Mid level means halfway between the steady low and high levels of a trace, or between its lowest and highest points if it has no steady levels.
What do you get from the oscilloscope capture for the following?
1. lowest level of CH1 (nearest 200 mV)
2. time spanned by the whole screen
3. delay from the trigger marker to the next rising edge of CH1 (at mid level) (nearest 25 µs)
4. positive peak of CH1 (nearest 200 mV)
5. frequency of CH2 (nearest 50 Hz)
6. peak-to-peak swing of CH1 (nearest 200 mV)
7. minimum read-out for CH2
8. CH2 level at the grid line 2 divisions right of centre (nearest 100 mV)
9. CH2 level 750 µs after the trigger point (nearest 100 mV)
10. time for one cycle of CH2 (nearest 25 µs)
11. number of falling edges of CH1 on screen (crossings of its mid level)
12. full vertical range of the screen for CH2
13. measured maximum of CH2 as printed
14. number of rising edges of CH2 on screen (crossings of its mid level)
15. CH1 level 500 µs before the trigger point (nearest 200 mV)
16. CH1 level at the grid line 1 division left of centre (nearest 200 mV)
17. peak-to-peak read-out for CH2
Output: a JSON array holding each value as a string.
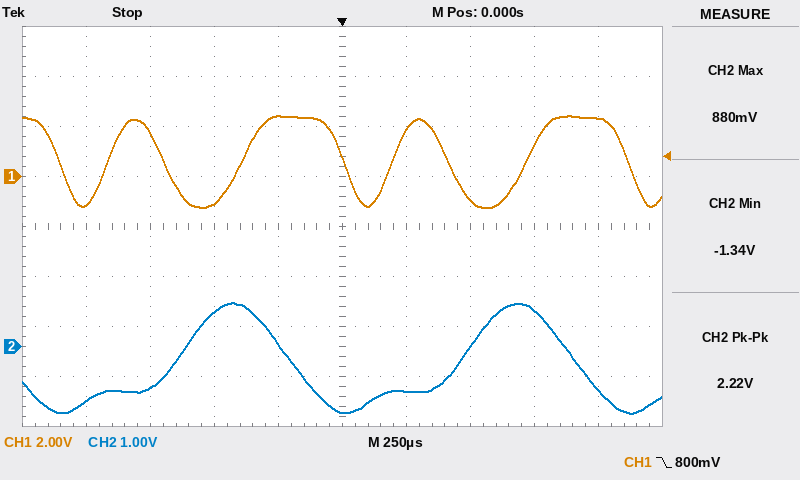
["-1.2 V", "2.5 ms", "200 µs", "2.4 V", "900 Hz", "3.6 V", "-1.34 V", "0.0 V", "700 mV", "1.100 ms", "5", "8 V", "880 mV", "2", "-1.0 V", "2.4 V", "2.22 V"]
